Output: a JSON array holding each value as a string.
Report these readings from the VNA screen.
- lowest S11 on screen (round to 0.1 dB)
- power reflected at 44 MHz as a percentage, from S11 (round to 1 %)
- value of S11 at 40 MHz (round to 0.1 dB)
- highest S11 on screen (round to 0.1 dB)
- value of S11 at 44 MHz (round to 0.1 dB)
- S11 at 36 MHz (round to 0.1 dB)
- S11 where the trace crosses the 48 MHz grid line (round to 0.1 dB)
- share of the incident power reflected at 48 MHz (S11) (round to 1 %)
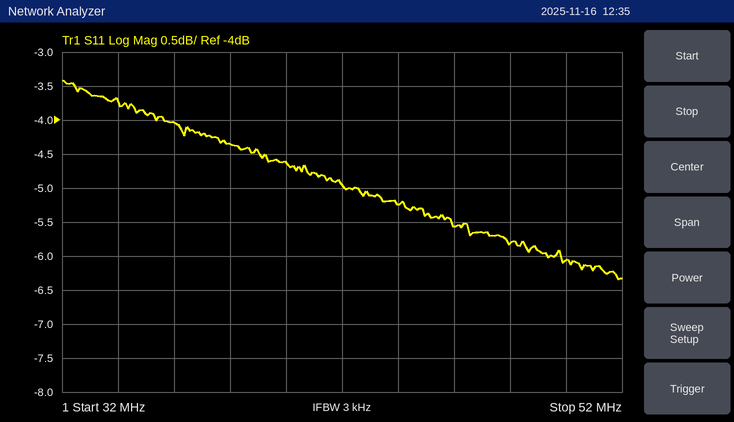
["-6.3 dB", "30 %", "-4.6 dB", "-3.4 dB", "-5.2 dB", "-4.0 dB", "-5.8 dB", "26 %"]
